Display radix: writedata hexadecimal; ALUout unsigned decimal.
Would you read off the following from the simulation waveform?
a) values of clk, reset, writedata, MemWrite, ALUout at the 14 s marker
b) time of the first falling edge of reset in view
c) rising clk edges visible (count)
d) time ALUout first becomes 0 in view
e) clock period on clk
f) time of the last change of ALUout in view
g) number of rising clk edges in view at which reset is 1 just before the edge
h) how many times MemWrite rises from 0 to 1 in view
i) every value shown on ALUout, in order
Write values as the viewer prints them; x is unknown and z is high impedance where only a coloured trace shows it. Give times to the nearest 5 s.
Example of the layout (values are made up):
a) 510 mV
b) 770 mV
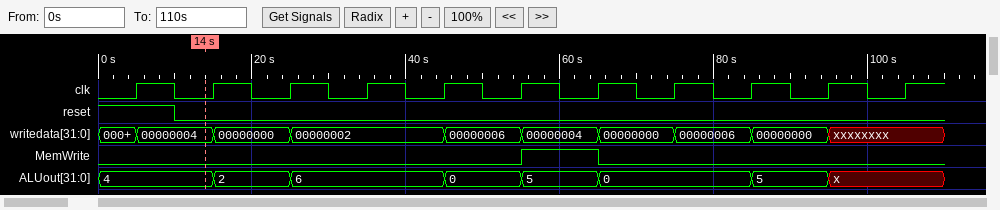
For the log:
a) clk=0, reset=0, writedata=00000004, MemWrite=0, ALUout=4
b) 10 s
c) 11
d) 45 s
e) 10 s
f) 95 s
g) 1
h) 1
i) 4, 2, 6, 0, 5, 0, 5, x
